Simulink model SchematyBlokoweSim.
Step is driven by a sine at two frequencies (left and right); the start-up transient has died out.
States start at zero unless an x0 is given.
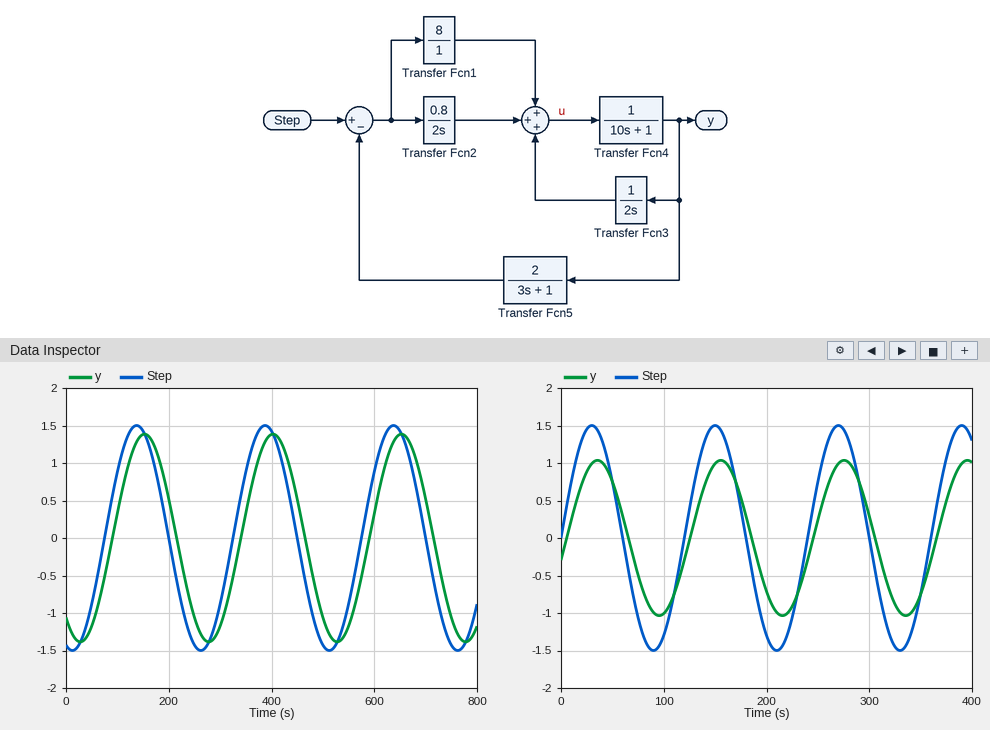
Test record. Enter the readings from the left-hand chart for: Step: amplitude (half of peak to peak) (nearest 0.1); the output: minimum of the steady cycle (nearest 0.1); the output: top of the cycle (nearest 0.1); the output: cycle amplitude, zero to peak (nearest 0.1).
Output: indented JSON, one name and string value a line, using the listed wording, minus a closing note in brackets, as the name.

{
  "Step: amplitude (half of peak to peak)": "1.5",
  "the output: minimum of the steady cycle": "-1.4",
  "the output: top of the cycle": "1.4",
  "the output: cycle amplitude, zero to peak": "1.4"
}
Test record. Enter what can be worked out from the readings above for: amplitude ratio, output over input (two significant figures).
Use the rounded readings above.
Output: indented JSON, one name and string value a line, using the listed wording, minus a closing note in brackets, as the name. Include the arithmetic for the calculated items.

{
  "amplitude ratio, output over input": "1.4 / 1.5 = 0.93"
}
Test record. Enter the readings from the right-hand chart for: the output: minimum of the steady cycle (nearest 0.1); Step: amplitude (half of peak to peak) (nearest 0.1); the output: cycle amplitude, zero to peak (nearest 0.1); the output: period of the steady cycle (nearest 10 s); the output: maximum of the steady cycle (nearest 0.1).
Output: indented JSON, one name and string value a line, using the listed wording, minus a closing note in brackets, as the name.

{
  "the output: minimum of the steady cycle": "-1.0",
  "Step: amplitude (half of peak to peak)": "1.5",
  "the output: cycle amplitude, zero to peak": "1.0",
  "the output: period of the steady cycle": "120 s",
  "the output: maximum of the steady cycle": "1.0"
}
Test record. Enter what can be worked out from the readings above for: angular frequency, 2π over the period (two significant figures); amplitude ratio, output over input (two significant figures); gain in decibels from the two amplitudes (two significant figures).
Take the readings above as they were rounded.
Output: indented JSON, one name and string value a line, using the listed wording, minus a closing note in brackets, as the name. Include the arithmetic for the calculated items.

{
  "angular frequency, 2π over the period": "2π / 120 = 0.052 rad/s",
  "amplitude ratio, output over input": "1 / 1.5 = 0.67",
  "gain in decibels from the two amplitudes": "20 log10(1 / 1.5) = -3.5 dB"
}
